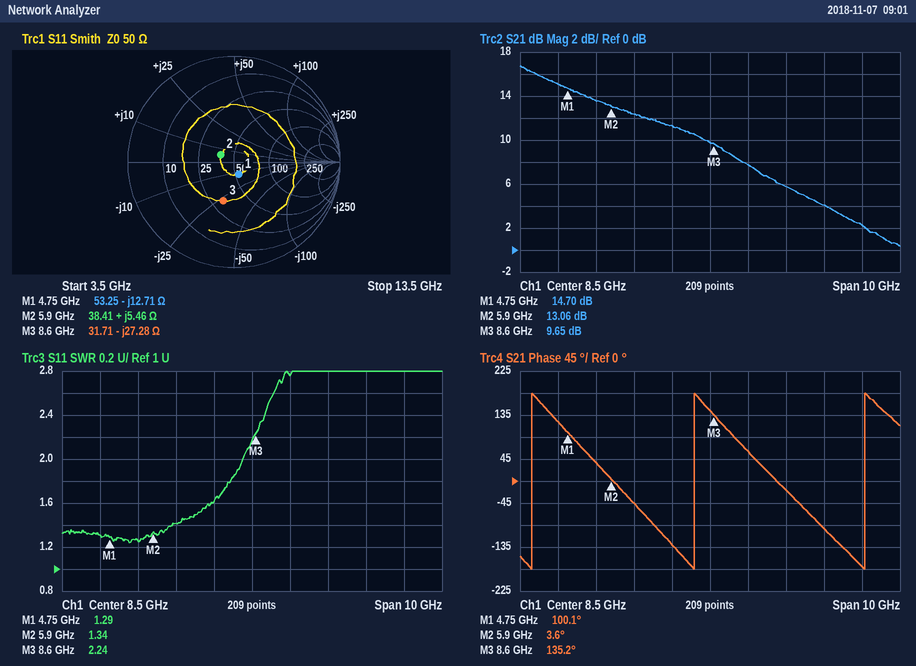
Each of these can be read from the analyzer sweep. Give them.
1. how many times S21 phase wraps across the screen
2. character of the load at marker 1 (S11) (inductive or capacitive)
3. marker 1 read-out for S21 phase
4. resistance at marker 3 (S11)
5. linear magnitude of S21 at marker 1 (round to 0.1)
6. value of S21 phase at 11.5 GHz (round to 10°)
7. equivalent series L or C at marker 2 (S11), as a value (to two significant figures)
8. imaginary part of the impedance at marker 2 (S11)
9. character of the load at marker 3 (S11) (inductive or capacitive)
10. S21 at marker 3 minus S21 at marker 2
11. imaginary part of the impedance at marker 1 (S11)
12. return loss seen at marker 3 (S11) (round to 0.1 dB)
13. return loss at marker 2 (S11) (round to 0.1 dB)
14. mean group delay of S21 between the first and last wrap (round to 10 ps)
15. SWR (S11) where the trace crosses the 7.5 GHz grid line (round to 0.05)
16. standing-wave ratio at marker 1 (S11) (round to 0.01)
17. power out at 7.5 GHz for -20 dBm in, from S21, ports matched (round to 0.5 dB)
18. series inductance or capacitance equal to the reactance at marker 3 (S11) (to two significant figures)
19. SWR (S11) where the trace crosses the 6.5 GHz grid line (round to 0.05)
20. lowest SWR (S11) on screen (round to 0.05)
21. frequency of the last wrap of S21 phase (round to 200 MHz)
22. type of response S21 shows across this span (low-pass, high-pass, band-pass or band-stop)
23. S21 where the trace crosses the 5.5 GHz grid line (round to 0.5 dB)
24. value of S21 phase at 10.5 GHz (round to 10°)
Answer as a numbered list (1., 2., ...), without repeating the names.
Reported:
1. 3
2. capacitive
3. 100.1°
4. 31.71 Ω
5. 5.4
6. -100°
7. 150 pH
8. +5.46 Ω
9. capacitive
10. -3.41 dB
11. -12.71 Ω
12. 8.4 dB
13. 16.8 dB
14. 230 ps
15. 1.60
16. 1.29
17. -8.5 dBm
18. 680 fF
19. 1.40
20. 1.25
21. 12.6 GHz
22. low-pass
23. 13.5 dB
24. -20°
